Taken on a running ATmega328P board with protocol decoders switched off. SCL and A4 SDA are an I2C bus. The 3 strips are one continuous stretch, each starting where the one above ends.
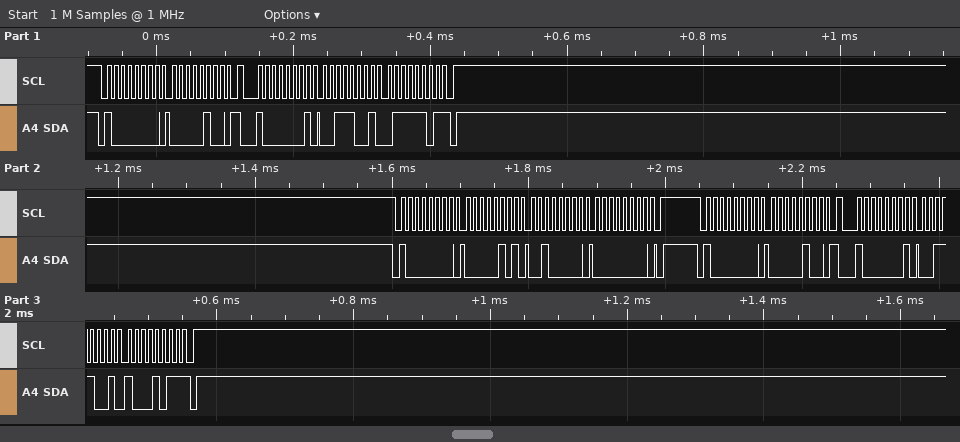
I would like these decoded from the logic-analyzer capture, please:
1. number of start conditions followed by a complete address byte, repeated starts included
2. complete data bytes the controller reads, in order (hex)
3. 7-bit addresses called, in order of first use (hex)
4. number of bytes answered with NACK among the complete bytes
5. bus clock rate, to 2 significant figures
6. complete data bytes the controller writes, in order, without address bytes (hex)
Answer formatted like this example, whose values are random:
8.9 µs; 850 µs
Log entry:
5; 39 7D 39 8B; 0x40; 2; 100 kHz; 04 05 20 00 04
